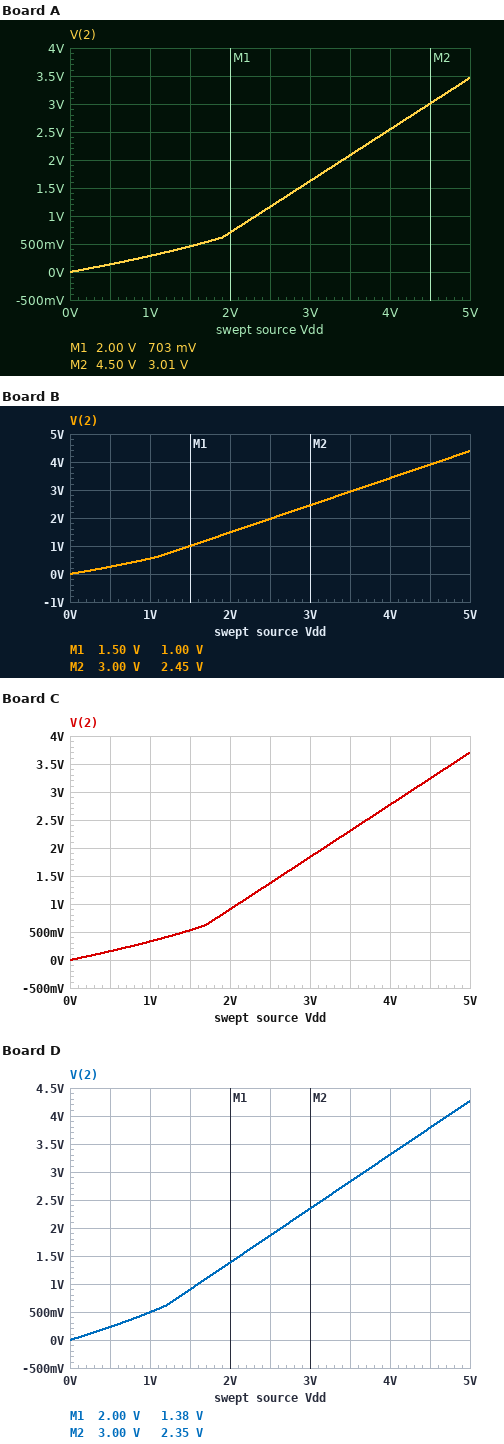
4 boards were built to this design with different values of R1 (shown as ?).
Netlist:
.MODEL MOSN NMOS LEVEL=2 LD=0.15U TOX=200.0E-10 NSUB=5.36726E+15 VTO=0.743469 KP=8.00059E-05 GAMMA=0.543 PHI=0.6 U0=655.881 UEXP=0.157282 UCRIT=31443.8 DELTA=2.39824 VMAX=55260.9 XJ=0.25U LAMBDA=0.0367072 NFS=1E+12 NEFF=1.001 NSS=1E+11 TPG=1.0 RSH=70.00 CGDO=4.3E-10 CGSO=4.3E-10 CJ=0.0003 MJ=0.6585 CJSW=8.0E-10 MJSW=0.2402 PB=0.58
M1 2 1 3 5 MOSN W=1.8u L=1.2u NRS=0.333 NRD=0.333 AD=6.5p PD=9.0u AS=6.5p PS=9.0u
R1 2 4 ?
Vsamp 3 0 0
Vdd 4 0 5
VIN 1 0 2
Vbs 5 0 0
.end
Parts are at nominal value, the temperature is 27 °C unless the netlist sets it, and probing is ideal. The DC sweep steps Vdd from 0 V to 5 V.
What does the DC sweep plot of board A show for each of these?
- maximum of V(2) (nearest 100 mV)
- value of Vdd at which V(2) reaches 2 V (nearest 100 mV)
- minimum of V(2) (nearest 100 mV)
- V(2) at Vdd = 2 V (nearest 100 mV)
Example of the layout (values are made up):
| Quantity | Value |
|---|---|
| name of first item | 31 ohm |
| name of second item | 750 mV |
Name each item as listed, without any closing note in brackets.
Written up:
| Quantity | Value |
|---|---|
| maximum of V(2) | 3.5 V |
| value of Vdd at which V(2) reaches 2 V | 3.4 V |
| minimum of V(2) | 0 V |
| V(2) at Vdd = 2 V | 700 mV |
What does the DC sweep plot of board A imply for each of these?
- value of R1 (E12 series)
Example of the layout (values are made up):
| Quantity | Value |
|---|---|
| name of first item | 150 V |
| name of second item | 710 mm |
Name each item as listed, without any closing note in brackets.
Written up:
| Quantity | Value |
|---|---|
| value of R1 | 18 kΩ |
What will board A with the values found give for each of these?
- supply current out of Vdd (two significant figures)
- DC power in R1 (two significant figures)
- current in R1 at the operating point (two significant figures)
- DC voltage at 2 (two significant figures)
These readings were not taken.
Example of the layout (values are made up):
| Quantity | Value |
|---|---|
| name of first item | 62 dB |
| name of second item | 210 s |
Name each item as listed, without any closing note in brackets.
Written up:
| Quantity | Value |
|---|---|
| supply current out of Vdd | 85 µA |
| DC power in R1 | 130 µW |
| current in R1 at the operating point | 85 µA |
| DC voltage at 2 | 3.5 V |
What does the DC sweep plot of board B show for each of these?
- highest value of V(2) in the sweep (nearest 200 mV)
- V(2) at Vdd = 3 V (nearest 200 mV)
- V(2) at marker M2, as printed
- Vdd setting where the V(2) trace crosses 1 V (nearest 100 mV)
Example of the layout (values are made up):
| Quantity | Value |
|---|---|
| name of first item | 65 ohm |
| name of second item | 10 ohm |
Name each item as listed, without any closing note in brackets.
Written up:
| Quantity | Value |
|---|---|
| highest value of V(2) in the sweep | 4.4 V |
| V(2) at Vdd = 3 V | 2.4 V |
| V(2) at marker M2, as printed | 2.45 V |
| Vdd setting where the V(2) trace crosses 1 V | 1.5 V |
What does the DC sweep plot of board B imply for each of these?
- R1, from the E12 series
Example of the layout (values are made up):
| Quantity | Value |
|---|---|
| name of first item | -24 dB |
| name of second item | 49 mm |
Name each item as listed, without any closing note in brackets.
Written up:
| Quantity | Value |
|---|---|
| R1, from the E12 series | 6.8 kΩ |
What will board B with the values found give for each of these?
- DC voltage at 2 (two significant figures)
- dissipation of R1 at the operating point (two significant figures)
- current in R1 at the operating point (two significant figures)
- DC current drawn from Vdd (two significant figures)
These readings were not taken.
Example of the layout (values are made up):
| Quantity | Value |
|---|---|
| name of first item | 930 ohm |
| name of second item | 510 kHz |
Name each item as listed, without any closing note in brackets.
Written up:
| Quantity | Value |
|---|---|
| DC voltage at 2 | 4.4 V |
| dissipation of R1 at the operating point | 55 µW |
| current in R1 at the operating point | 90 µA |
| DC current drawn from Vdd | 90 µA |
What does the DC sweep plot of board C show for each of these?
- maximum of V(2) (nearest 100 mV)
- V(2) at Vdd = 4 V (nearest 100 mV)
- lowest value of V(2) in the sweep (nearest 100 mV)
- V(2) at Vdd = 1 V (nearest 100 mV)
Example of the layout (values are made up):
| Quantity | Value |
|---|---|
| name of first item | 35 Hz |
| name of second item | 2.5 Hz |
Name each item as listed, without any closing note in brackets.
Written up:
| Quantity | Value |
|---|---|
| maximum of V(2) | 3.7 V |
| V(2) at Vdd = 4 V | 2.8 V |
| lowest value of V(2) in the sweep | 0 V |
| V(2) at Vdd = 1 V | 300 mV |
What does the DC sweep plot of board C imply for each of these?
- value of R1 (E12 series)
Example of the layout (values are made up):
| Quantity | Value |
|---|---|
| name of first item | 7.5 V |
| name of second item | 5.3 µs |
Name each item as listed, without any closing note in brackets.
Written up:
| Quantity | Value |
|---|---|
| value of R1 | 15 kΩ |
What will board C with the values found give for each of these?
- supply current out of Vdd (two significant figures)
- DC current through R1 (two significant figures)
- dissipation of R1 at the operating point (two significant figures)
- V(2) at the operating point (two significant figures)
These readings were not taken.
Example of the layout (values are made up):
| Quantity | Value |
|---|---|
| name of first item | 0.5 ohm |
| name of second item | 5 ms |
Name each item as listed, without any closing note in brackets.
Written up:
| Quantity | Value |
|---|---|
| supply current out of Vdd | 86 µA |
| DC current through R1 | 86 µA |
| dissipation of R1 at the operating point | 110 µW |
| V(2) at the operating point | 3.7 V |
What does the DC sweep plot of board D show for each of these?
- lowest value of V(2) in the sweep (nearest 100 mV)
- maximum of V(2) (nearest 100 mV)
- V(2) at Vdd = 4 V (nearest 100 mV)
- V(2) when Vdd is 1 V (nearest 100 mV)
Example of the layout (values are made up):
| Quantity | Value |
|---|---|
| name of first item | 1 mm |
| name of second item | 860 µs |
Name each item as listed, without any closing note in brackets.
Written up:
| Quantity | Value |
|---|---|
| lowest value of V(2) in the sweep | 0 V |
| maximum of V(2) | 4.3 V |
| V(2) at Vdd = 4 V | 3.3 V |
| V(2) when Vdd is 1 V | 500 mV |
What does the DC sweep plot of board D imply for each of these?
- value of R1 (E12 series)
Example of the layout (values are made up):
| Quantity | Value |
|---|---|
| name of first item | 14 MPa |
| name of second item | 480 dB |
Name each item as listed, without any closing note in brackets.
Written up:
| Quantity | Value |
|---|---|
| value of R1 | 8.2 kΩ |
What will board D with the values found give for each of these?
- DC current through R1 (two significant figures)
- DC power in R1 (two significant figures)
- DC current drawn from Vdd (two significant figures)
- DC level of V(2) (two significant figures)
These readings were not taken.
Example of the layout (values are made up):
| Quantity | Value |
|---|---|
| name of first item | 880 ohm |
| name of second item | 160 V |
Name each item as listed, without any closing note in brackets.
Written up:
| Quantity | Value |
|---|---|
| DC current through R1 | 89 µA |
| DC power in R1 | 65 µW |
| DC current drawn from Vdd | 89 µA |
| DC level of V(2) | 4.3 V |
